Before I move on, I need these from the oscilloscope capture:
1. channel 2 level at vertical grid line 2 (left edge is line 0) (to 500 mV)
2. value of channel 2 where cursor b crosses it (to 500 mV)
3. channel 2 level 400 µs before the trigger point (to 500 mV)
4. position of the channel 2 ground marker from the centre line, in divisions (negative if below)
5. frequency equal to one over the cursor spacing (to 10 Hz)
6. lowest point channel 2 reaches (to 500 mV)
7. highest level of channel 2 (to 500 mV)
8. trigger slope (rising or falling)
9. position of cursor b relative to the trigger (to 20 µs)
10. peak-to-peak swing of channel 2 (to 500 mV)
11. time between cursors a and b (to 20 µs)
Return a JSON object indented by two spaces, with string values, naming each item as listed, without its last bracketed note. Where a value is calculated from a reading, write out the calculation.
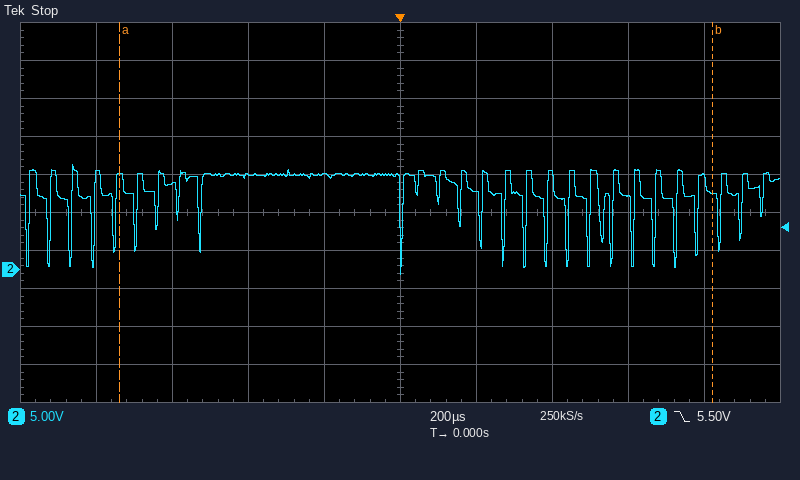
{
  "channel 2 level at vertical grid line 2 (left edge is line 0)": "11.0 V",
  "value of channel 2 where cursor b crosses it": "10.0 V",
  "channel 2 level 400 µs before the trigger point": "12.5 V",
  "position of the channel 2 ground marker from the centre line, in divisions": "-1.5 div",
  "frequency equal to one over the cursor spacing": "1 / 1.56 ms ≈ 640 Hz",
  "lowest point channel 2 reaches": "-500 mV",
  "highest level of channel 2": "14.0 V",
  "trigger slope": "falling",
  "position of cursor b relative to the trigger": "+820 µs",
  "peak-to-peak swing of channel 2": "14.0 V − (-500 mV) = 14.5 V",
  "time between cursors a and b": "1.56 ms"
}
